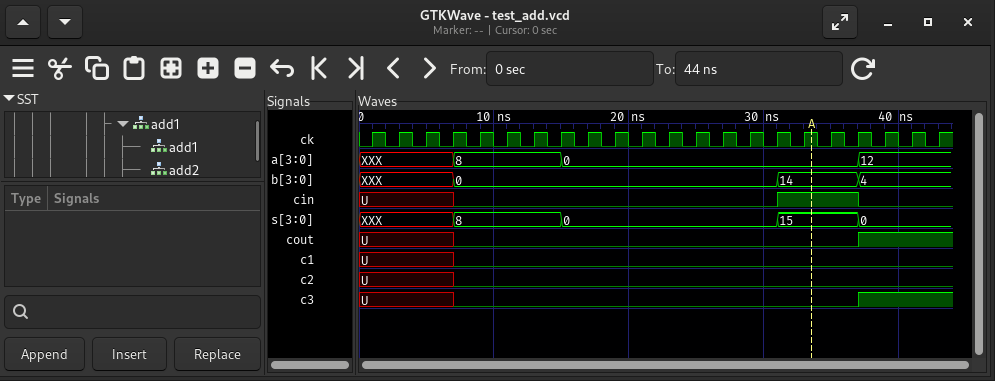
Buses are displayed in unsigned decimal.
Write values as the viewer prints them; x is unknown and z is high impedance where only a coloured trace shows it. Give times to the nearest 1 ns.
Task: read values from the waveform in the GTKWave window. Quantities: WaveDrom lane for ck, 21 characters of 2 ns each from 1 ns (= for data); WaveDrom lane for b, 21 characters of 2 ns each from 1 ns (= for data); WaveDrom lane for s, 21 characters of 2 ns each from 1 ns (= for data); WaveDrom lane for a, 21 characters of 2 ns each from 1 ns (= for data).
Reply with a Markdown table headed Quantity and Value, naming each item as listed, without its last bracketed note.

| Quantity | Value |
|---|---|
| WaveDrom lane for ck, 21 characters of 2 ns each from 1 ns | {name: 'ck', wave: 'p....................'} |
| WaveDrom lane for b, 21 characters of 2 ns each from 1 ns | {name: 'b', wave: 'x..=...........=..=..', data: '0 14 4'} |
| WaveDrom lane for s, 21 characters of 2 ns each from 1 ns | {name: 's', wave: 'x..=...=.......=..=..', data: '8 0 15 0'} |
| WaveDrom lane for a, 21 characters of 2 ns each from 1 ns | {name: 'a', wave: 'x..=...=..........=..', data: '8 0 12'} |
